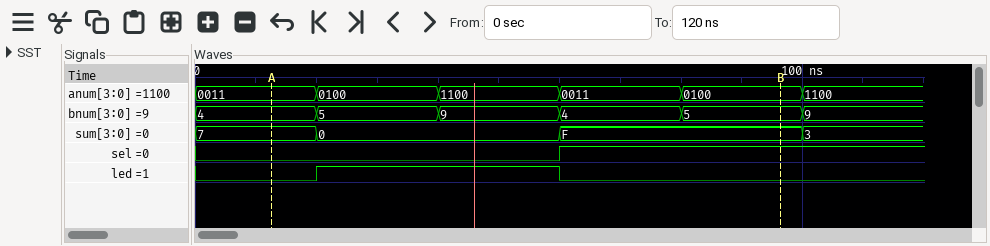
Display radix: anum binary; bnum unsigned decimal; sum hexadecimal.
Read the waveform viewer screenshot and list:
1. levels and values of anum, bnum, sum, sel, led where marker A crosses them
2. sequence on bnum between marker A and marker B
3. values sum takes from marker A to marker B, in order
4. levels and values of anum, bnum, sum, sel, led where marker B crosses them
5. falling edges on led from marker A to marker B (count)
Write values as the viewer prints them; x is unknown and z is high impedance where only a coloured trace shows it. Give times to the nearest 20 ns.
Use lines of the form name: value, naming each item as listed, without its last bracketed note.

levels and values of anum, bnum, sum, sel, led where marker A crosses them: anum=0011, bnum=4, sum=7, sel=0, led=0
sequence on bnum between marker A and marker B: 4, 5, 9, 4, 5
values sum takes from marker A to marker B, in order: 7, 0, F
levels and values of anum, bnum, sum, sel, led where marker B crosses them: anum=0100, bnum=5, sum=F, sel=1, led=0
falling edges on led from marker A to marker B: 1
